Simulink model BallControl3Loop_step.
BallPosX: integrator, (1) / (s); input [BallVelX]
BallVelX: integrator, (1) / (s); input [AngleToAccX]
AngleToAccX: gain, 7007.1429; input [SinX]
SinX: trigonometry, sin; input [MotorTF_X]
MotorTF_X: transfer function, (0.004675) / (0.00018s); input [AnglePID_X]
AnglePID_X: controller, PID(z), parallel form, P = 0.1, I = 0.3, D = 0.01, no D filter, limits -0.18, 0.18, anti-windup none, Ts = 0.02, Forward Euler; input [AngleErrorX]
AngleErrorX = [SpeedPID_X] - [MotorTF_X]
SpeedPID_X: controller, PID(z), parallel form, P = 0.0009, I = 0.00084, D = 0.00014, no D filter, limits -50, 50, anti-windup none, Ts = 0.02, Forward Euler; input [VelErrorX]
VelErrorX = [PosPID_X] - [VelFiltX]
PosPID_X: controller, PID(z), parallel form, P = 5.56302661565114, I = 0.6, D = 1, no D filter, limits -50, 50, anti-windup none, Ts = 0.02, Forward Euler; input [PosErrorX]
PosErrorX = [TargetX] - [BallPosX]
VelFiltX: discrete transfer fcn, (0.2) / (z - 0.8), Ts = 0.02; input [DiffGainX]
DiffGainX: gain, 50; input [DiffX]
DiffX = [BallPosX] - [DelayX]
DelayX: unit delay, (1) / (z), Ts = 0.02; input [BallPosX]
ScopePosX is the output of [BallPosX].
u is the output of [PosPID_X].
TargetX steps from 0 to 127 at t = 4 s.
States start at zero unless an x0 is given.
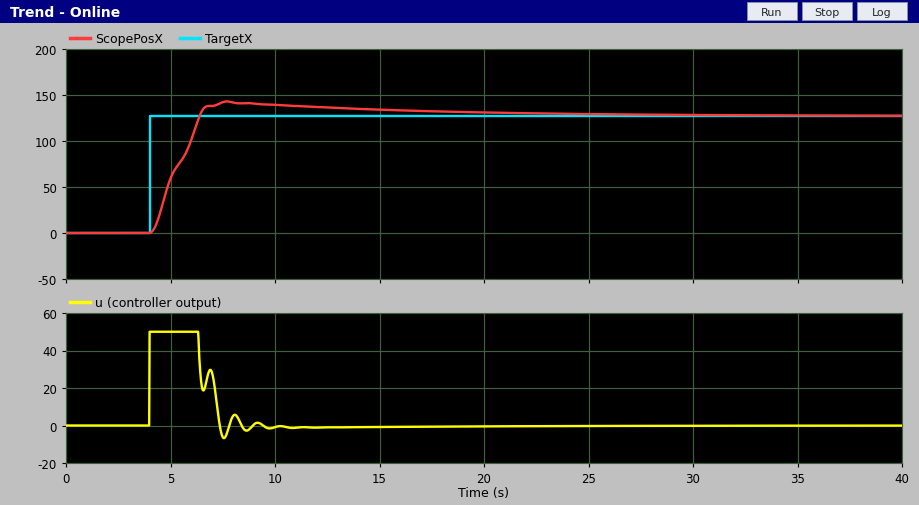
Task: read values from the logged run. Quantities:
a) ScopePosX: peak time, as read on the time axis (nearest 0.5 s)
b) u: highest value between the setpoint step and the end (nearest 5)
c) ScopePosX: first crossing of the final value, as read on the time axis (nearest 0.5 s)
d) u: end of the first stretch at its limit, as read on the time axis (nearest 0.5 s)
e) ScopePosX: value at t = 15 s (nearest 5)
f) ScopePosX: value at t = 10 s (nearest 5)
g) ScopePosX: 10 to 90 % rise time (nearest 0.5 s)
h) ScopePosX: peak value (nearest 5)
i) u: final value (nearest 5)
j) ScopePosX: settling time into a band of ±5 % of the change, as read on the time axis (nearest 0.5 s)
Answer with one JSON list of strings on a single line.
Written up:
["7.5 s", "50", "6.5 s", "6.5 s", "135", "140", "2.0 s", "145", "0", "16.0 s"]
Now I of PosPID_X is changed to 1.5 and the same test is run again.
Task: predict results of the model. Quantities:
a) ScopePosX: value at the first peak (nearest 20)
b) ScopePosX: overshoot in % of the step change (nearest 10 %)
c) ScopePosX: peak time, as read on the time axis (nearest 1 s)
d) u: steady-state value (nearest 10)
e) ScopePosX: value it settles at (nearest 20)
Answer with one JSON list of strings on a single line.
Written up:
["160", "30 %", "7 s", "0", "120"]
